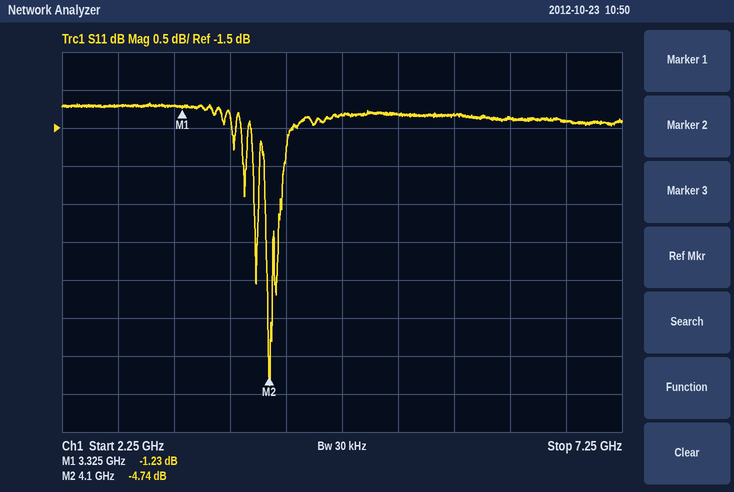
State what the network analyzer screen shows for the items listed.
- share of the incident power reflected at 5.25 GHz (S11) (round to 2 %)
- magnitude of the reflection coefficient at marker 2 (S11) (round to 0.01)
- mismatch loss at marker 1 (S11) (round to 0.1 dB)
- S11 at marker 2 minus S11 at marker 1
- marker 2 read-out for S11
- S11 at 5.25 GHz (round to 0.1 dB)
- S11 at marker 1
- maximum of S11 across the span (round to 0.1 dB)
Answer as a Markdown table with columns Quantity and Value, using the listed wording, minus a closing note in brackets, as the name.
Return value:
| Quantity | Value |
|---|---|
| share of the incident power reflected at 5.25 GHz (S11) | 74 % |
| magnitude of the reflection coefficient at marker 2 (S11) | 0.58 |
| mismatch loss at marker 1 (S11) | 6.1 dB |
| S11 at marker 2 minus S11 at marker 1 | -3.51 dB |
| marker 2 read-out for S11 | -4.74 dB |
| S11 at 5.25 GHz | -1.3 dB |
| S11 at marker 1 | -1.23 dB |
| maximum of S11 across the span | -1.2 dB |
